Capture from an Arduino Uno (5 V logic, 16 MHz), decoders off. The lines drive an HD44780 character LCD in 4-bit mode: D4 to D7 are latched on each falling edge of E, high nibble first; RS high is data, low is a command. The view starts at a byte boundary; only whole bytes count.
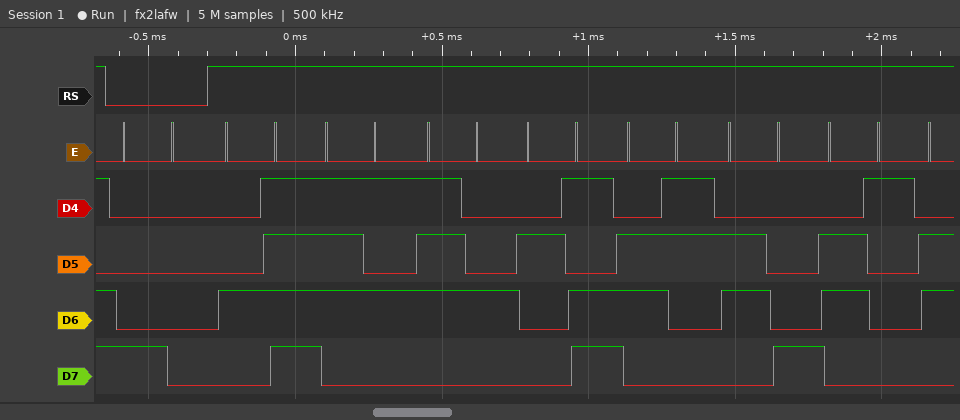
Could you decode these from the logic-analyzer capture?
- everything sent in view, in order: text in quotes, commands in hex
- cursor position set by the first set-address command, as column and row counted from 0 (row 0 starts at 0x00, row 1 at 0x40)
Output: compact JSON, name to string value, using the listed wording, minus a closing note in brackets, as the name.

{"everything sent in view, in order: text in quotes, commands in hex": "0x80 \"Out-cha\"", "cursor position set by the first set-address command, as column and row counted from 0": "column 0, row 0"}
